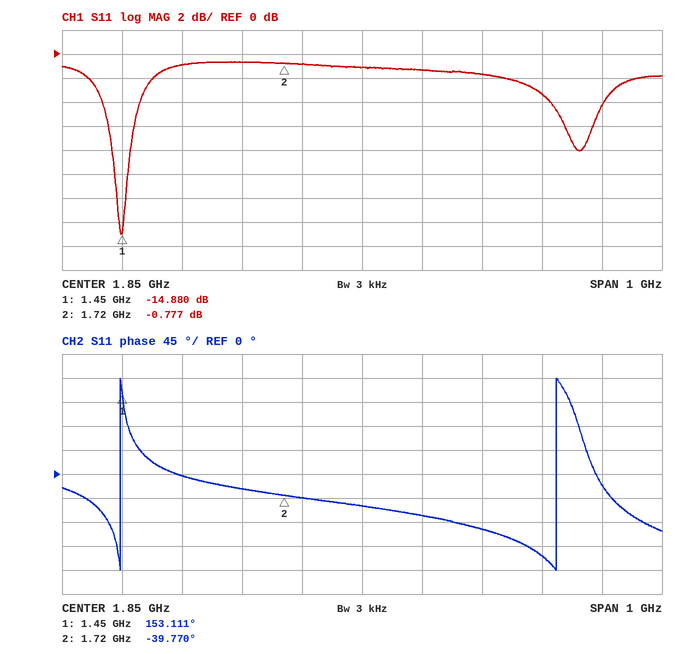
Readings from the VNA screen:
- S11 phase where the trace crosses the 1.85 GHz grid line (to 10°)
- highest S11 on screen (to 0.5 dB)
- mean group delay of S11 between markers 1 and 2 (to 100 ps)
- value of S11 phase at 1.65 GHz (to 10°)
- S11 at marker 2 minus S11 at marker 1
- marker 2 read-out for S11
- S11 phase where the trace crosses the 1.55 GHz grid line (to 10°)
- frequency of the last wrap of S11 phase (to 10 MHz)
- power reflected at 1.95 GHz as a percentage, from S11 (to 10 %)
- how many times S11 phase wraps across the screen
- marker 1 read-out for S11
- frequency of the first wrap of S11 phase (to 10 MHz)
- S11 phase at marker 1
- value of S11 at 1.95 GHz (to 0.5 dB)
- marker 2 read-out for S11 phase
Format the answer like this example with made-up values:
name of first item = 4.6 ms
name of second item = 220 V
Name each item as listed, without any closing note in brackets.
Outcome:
S11 phase where the trace crosses the 1.85 GHz grid line = -60°
highest S11 on screen = -0.5 dB
mean group delay of S11 between markers 1 and 2 = 2.0 ns
value of S11 phase at 1.65 GHz = -30°
S11 at marker 2 minus S11 at marker 1 = 14.103 dB
marker 2 read-out for S11 = -0.777 dB
S11 phase where the trace crosses the 1.55 GHz grid line = 0°
frequency of the last wrap of S11 phase = 2.17 GHz
power reflected at 1.95 GHz as a percentage, from S11 = 70 %
how many times S11 phase wraps across the screen = 2
marker 1 read-out for S11 = -14.880 dB
frequency of the first wrap of S11 phase = 1.45 GHz
S11 phase at marker 1 = 153.111°
value of S11 at 1.95 GHz = -1.5 dB
marker 2 read-out for S11 phase = -39.770°
